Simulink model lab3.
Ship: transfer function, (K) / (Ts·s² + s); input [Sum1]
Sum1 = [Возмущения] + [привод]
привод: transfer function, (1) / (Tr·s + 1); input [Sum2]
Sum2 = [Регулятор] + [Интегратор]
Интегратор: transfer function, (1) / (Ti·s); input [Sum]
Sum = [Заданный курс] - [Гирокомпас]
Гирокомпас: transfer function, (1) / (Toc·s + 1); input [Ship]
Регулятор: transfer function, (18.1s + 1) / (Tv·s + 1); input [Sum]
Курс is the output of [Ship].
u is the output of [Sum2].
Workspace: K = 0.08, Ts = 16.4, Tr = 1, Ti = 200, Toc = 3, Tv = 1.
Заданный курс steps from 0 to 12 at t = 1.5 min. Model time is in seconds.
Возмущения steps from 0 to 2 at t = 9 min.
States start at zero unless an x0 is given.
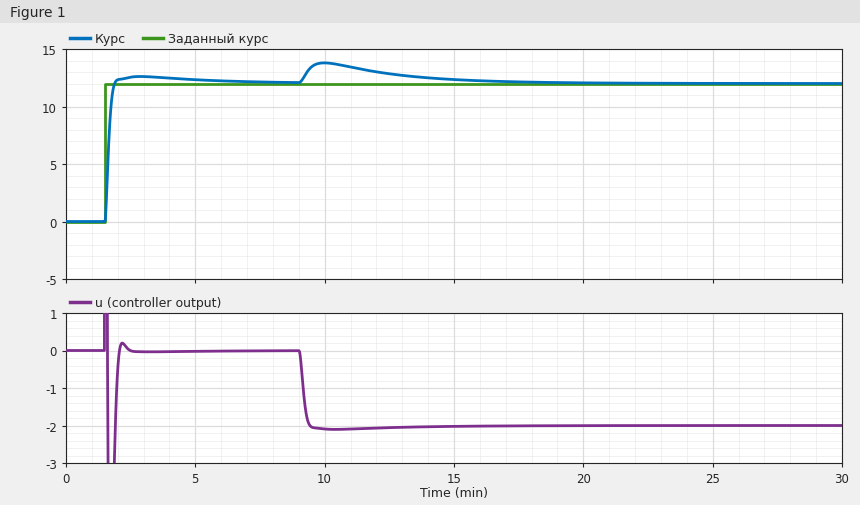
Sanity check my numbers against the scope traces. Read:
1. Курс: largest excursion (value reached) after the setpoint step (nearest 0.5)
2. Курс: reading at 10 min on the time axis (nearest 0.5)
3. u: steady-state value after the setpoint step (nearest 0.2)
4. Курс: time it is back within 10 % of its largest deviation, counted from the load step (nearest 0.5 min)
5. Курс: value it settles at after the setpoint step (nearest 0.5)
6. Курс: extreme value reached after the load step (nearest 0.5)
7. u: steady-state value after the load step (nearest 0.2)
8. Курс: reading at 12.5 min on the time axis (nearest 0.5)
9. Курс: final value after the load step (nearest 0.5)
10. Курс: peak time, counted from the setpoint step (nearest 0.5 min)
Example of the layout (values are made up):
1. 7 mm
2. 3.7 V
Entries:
1. 12.5
2. 14.0
3. 0.0
4. 8.0 min
5. 12.0
6. 14.0
7. -2.0
8. 13.0
9. 12.0
10. 1.5 min
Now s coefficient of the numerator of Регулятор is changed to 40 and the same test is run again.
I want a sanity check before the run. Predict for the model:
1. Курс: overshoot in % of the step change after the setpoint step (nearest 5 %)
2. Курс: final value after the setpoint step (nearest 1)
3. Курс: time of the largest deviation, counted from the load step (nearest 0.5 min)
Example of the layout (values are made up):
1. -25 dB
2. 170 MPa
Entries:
1. 15 %
2. 12
3. 1.5 min
